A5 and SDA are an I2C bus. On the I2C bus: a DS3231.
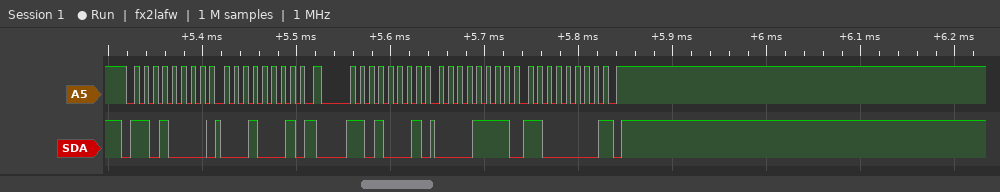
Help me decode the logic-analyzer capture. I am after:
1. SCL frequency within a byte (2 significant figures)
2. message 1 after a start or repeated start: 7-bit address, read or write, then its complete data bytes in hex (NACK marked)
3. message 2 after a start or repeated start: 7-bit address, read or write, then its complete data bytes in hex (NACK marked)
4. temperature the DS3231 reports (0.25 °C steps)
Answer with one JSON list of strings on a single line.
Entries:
["100 kHz", "0x68 write: 11", "0x68 read: 0F C0 NACK", "15.75 °C"]
